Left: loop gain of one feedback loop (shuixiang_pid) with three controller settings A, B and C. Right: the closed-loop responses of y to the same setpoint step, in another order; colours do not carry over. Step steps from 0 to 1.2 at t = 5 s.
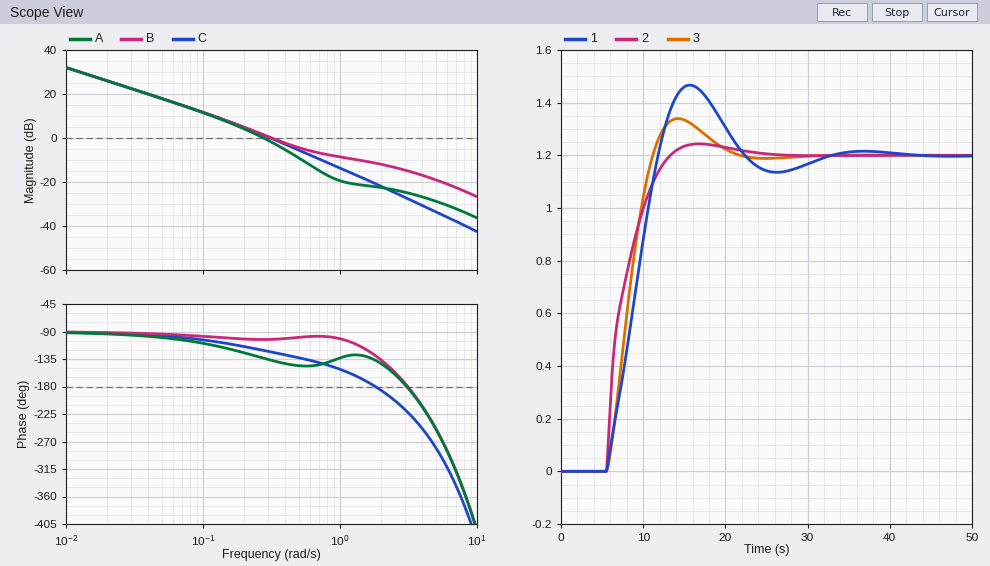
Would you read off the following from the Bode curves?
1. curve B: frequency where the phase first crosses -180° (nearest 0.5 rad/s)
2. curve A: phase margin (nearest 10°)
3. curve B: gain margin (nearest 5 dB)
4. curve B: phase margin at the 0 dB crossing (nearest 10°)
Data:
3.0 rad/s
50°
15 dB
80°
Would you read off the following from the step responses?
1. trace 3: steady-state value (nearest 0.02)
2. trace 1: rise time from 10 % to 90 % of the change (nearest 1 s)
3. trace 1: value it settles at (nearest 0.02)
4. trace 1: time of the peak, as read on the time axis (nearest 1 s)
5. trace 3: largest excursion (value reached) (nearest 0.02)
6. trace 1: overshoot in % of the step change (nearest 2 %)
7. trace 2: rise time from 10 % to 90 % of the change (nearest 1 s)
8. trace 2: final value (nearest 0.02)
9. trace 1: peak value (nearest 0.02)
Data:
1.20
5 s
1.20
16 s
1.34
22 %
5 s
1.20
1.46
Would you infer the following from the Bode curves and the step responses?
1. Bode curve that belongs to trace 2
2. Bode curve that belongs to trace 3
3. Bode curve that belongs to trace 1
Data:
B
C
A
